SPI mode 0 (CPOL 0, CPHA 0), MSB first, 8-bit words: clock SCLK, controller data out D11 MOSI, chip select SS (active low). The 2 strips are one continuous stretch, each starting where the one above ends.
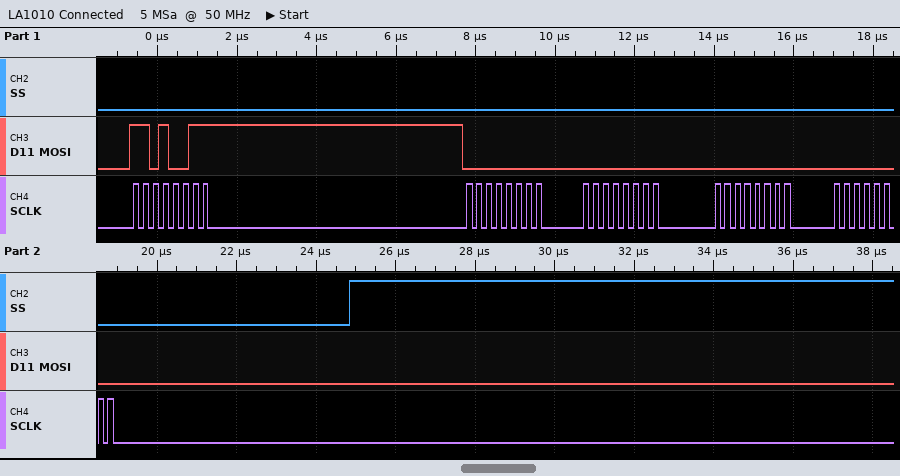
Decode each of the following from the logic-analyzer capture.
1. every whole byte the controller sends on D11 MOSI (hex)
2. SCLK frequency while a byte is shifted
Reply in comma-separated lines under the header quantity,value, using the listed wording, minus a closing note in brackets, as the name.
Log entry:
quantity,value
every whole byte the controller sends on D11 MOSI,D3 00 00 00 00
SCLK frequency while a byte is shifted,4 MHz
